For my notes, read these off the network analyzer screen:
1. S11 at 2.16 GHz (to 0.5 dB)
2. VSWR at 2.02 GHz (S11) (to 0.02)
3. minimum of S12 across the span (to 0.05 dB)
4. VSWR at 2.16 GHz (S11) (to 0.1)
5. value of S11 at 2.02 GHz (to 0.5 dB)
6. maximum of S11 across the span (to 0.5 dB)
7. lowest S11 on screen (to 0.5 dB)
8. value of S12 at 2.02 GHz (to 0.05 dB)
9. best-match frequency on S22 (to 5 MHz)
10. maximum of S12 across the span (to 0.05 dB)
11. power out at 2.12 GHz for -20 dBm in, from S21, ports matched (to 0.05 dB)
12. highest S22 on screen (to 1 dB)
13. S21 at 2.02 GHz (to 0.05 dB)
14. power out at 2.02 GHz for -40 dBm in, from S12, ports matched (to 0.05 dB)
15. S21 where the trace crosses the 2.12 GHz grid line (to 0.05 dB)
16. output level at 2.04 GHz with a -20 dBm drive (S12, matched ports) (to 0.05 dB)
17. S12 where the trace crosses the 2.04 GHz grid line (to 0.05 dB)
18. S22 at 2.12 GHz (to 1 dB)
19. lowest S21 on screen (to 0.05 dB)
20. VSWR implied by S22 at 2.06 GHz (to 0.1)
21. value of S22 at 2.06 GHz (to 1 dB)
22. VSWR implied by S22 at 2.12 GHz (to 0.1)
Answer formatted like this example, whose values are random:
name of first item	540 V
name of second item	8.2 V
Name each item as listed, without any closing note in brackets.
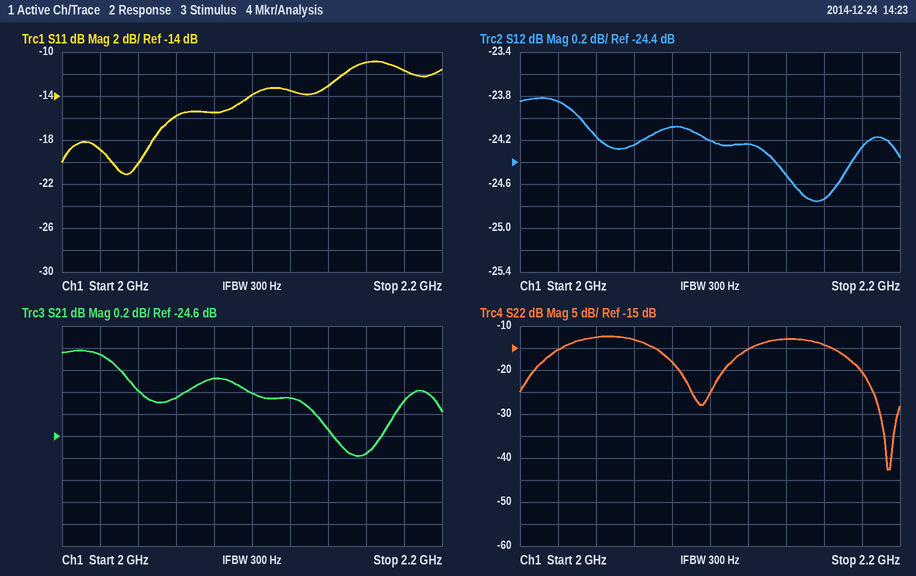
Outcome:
S11 at 2.16 GHz	-11.0 dB
VSWR at 2.02 GHz (S11)	1.26
minimum of S12 across the span	-24.75 dB
VSWR at 2.16 GHz (S11)	1.8
value of S11 at 2.02 GHz	-19.0 dB
maximum of S11 across the span	-11.0 dB
lowest S11 on screen	-21.0 dB
value of S12 at 2.02 GHz	-23.85 dB
best-match frequency on S22	2.195 GHz
maximum of S12 across the span	-23.80 dB
power out at 2.12 GHz for -20 dBm in, from S21, ports matched	-44.25 dBm
highest S22 on screen	-12 dB
S21 at 2.02 GHz	-23.85 dB
power out at 2.02 GHz for -40 dBm in, from S12, ports matched	-63.85 dBm
S21 where the trace crosses the 2.12 GHz grid line	-24.25 dB
output level at 2.04 GHz with a -20 dBm drive (S12, matched ports)	-44.15 dBm
S12 where the trace crosses the 2.04 GHz grid line	-24.15 dB
S22 at 2.12 GHz	-15 dB
lowest S21 on screen	-24.80 dB
VSWR implied by S22 at 2.06 GHz	1.6
value of S22 at 2.06 GHz	-13 dB
VSWR implied by S22 at 2.12 GHz	1.4
